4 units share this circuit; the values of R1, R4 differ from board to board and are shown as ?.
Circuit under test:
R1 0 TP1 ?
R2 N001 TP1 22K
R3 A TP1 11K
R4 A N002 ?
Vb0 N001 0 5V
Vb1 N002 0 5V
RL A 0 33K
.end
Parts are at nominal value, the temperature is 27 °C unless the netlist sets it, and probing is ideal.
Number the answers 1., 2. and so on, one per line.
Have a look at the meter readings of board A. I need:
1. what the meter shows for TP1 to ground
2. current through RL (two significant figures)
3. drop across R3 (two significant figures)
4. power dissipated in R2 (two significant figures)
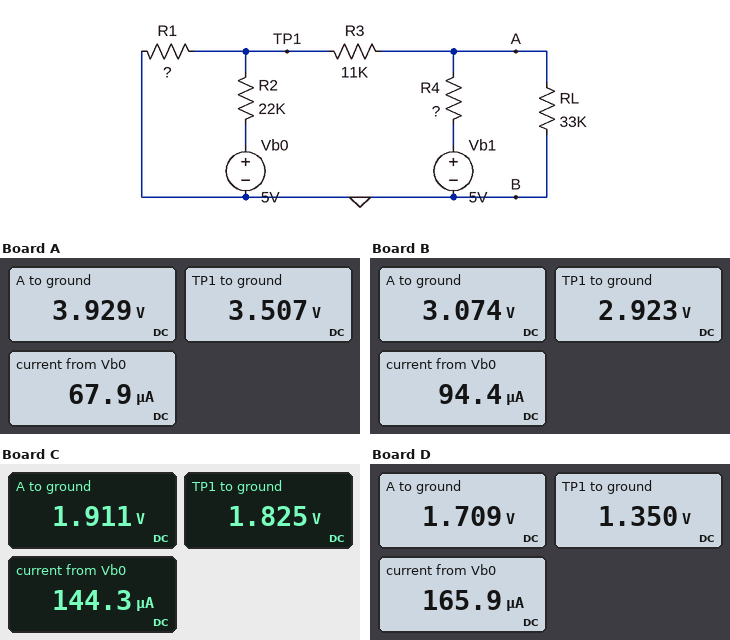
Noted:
1. 3.507 V
2. 120 µA
3. 420 mV
4. 100 µW
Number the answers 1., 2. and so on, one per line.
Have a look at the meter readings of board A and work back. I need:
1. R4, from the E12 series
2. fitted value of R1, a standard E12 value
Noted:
1. 6.8 kΩ
2. 33 kΩ
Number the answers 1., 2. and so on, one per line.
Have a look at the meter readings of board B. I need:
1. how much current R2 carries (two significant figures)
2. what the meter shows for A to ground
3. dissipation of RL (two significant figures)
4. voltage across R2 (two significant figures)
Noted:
1. 94 µA
2. 3.074 V
3. 290 µW
4. 2.1 V
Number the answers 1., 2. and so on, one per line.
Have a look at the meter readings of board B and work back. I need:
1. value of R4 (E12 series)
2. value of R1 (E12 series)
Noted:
1. 18 kΩ
2. 27 kΩ
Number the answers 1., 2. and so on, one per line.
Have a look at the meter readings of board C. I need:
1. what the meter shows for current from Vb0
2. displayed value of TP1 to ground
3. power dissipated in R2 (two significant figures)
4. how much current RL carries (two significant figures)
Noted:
1. 144.3 µA
2. 1.825 V
3. 460 µW
4. 58 µA
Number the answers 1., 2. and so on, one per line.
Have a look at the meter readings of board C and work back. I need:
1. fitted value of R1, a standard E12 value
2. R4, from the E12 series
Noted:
1. 12 kΩ
2. 47 kΩ
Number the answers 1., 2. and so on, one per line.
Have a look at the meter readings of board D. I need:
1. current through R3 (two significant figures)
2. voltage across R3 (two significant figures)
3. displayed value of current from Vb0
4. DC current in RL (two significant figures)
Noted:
1. 33 µA
2. 360 mV
3. 165.9 µA
4. 52 µA
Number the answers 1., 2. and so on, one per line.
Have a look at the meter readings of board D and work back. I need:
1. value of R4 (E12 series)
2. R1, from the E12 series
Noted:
1. 39 kΩ
2. 6.8 kΩ
